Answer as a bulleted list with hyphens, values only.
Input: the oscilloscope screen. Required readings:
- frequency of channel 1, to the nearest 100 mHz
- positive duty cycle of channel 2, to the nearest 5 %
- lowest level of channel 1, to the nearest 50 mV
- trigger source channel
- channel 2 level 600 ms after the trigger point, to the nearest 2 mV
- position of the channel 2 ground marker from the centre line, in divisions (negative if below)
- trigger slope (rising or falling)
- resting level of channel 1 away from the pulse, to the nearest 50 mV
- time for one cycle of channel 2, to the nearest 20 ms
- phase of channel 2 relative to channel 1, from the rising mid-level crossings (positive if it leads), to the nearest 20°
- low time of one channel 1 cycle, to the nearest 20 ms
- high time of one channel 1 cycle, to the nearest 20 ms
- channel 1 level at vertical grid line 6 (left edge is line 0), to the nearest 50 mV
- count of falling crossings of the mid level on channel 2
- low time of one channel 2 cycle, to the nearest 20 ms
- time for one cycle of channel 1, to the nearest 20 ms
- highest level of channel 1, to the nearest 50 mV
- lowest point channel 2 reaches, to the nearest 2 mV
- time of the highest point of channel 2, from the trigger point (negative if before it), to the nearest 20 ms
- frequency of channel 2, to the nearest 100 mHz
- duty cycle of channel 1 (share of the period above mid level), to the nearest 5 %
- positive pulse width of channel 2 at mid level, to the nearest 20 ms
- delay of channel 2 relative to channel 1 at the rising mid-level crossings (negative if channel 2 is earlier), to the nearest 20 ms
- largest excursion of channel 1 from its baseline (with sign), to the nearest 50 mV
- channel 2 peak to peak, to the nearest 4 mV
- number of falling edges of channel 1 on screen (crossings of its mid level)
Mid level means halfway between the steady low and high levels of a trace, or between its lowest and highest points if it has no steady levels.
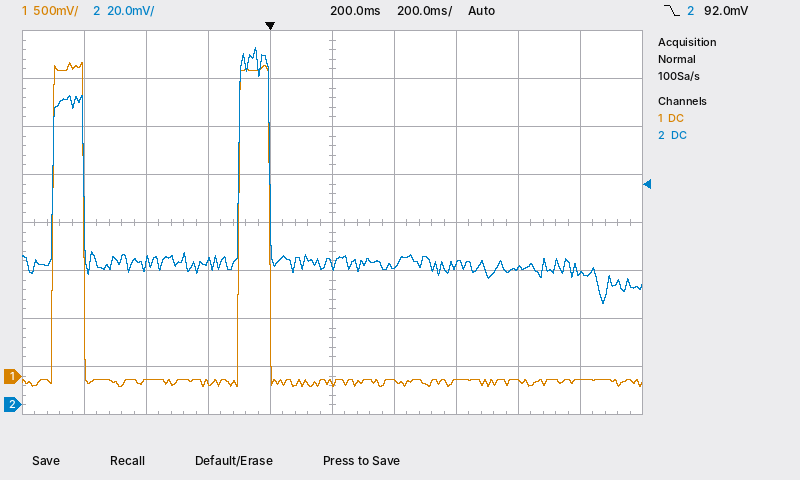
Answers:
- 1.7 Hz
- 15 %
- -100 mV
- channel 2
- 58 mV
- -3.8 div
- falling
- -50 mV
- 600 ms
- 0°
- 500 ms
- 100 ms
- -50 mV
- 2
- 500 ms
- 600 ms
- 3.25 V
- 42 mV
- -40 ms
- 1.7 Hz
- 15 %
- 100 ms
- 0 ms
- +3.30 V
- 108 mV
- 2
